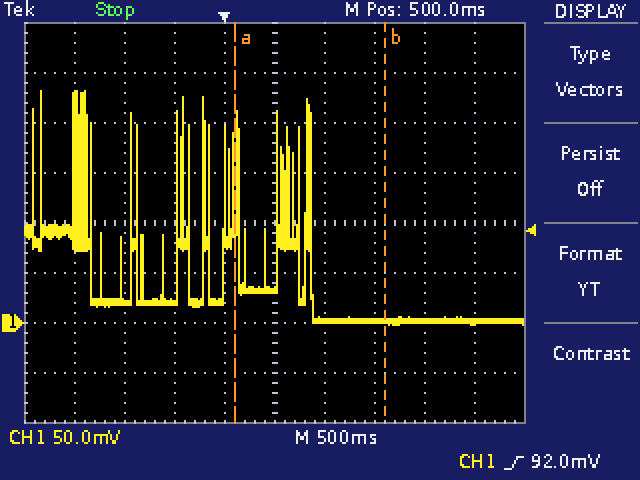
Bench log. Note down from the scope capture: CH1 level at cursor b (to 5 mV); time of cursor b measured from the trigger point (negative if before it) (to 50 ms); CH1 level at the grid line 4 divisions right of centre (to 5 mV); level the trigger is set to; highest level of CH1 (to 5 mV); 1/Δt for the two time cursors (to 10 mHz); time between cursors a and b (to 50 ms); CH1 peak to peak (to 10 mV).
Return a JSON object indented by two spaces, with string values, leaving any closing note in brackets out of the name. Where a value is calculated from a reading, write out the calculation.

{
  "CH1 level at cursor b": "0 mV",
  "time of cursor b measured from the trigger point (negative if before it)": "+1.60 s",
  "CH1 level at the grid line 4 divisions right of centre": "0 mV",
  "level the trigger is set to": "92.0 mV",
  "highest level of CH1": "230 mV",
  "1/Δt for the two time cursors": "1 / 1.50 s ≈ 670 mHz",
  "time between cursors a and b": "1.50 s",
  "CH1 peak to peak": "230 mV"
}
